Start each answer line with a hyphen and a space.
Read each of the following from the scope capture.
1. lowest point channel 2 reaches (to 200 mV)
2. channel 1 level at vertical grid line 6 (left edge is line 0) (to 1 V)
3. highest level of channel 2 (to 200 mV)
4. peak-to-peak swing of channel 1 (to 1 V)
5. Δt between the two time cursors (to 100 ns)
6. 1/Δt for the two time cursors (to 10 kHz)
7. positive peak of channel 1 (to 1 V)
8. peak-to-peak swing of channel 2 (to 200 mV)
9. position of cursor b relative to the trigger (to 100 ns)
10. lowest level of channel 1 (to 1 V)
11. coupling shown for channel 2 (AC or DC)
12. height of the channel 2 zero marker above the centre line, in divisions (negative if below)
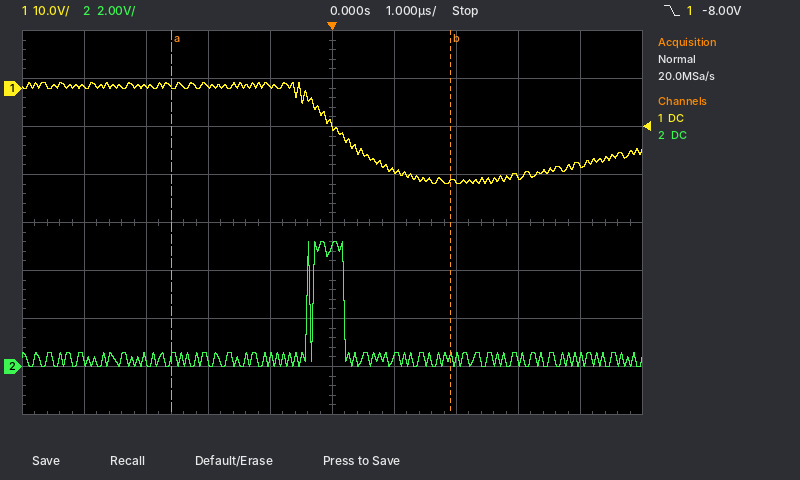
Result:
- 0.0 V
- -17 V
- 5.2 V
- 21 V
- 4.5 µs
- 220 kHz
- 1 V
- 5.2 V
- +1.9 µs
- -20 V
- DC
- -3.0 div
